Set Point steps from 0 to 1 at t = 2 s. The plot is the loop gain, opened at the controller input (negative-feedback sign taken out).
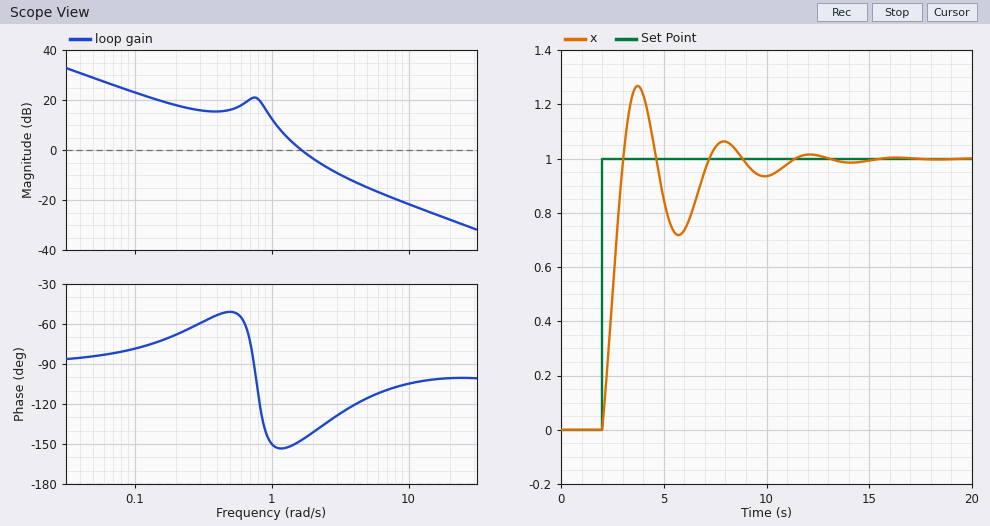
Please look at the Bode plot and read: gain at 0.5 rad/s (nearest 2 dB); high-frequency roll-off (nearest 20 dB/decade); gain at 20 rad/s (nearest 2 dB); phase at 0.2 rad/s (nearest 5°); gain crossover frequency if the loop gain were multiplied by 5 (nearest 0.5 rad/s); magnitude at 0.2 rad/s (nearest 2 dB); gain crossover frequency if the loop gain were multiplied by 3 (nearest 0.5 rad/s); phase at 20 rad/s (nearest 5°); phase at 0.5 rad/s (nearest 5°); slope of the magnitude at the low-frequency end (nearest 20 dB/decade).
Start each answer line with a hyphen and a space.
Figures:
- 16 dB
- -20 dB/decade
- -28 dB
- -70°
- 4.5 rad/s
- 18 dB
- 3.0 rad/s
- -100°
- -50°
- -20 dB/decade
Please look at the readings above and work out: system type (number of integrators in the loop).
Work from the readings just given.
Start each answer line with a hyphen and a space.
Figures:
- 1
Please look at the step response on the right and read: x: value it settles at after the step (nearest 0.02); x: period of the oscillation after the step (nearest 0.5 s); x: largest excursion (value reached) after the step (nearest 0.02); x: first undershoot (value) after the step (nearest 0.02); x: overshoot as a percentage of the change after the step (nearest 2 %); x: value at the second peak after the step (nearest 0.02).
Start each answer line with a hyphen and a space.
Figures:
- 1.00
- 4.0 s
- 1.26
- 0.72
- 26 %
- 1.06
